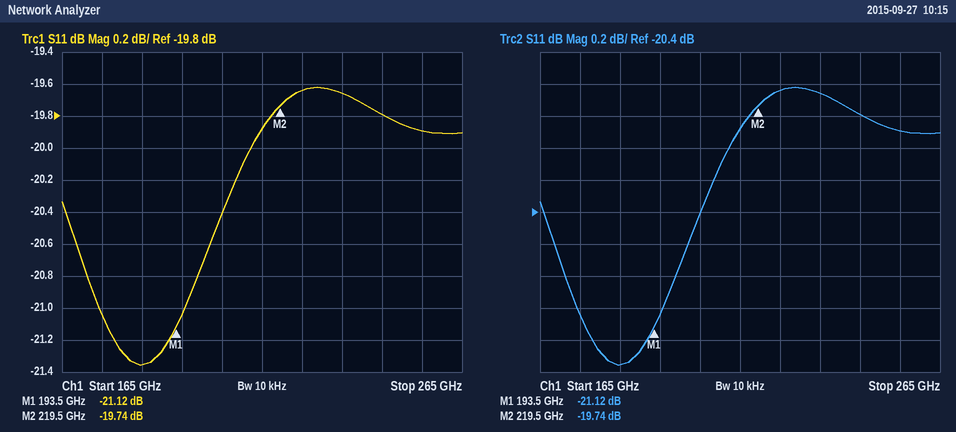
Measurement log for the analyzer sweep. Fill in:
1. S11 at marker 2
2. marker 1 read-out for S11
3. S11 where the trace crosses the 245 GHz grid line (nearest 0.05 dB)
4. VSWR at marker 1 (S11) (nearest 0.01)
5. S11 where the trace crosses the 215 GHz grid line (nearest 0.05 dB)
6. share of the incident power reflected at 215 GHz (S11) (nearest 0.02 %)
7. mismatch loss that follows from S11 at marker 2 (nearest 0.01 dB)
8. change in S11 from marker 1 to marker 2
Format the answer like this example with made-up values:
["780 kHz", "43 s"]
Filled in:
["-19.74 dB", "-21.12 dB", "-19.80 dB", "1.19", "-19.90 dB", "1.02 %", "0.05 dB", "1.38 dB"]
